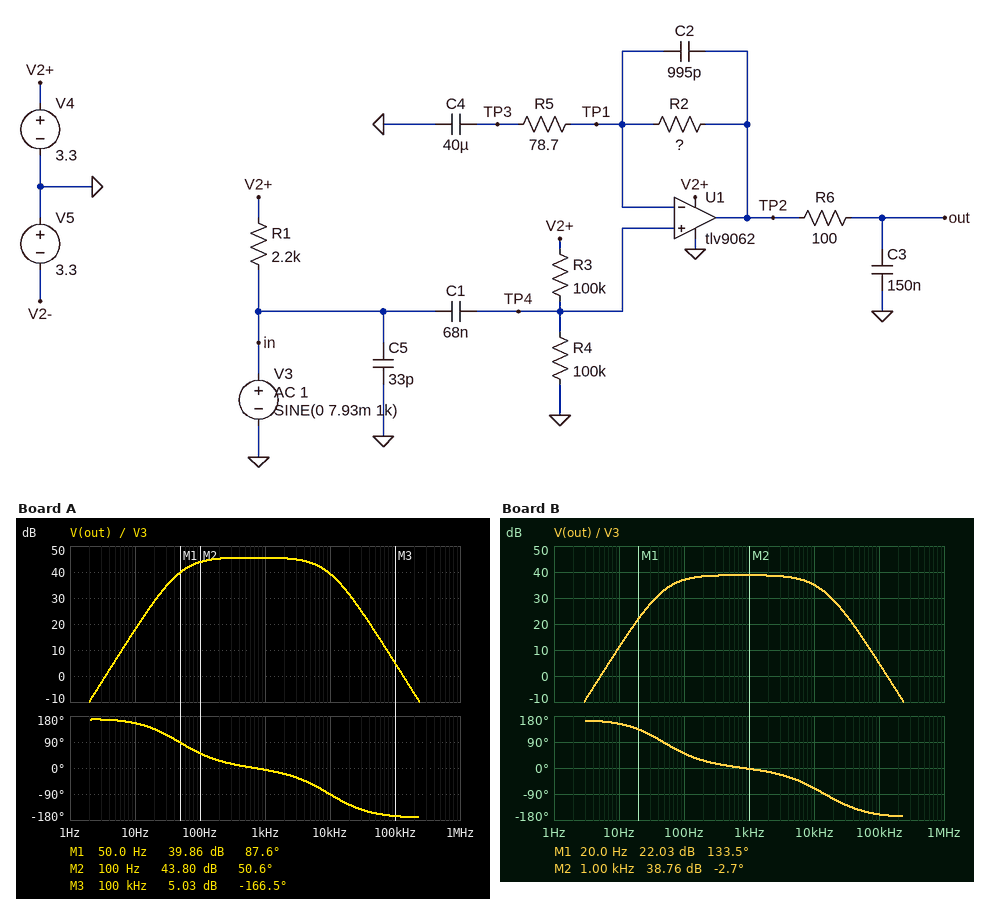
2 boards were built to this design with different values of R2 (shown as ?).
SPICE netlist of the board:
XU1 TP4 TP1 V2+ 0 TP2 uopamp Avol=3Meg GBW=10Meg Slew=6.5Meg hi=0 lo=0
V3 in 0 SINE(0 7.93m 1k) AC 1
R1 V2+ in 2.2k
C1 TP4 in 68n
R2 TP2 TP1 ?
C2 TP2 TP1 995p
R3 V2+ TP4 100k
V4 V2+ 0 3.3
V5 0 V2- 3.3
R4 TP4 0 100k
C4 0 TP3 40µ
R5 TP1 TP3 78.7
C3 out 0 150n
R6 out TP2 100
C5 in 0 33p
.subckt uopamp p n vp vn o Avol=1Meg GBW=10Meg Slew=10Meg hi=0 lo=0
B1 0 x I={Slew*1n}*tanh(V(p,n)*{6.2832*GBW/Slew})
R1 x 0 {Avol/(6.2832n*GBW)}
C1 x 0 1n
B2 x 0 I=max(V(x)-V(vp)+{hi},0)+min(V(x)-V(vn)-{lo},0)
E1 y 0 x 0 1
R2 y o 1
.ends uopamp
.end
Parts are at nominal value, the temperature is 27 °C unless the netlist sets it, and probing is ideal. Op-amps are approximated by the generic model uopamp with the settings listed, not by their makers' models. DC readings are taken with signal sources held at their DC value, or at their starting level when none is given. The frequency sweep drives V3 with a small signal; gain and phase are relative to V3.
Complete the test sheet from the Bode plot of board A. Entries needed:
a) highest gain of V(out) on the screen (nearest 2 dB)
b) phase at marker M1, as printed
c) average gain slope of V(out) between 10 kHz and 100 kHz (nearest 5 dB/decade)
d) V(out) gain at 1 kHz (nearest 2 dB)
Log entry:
46 dB
87.6 deg
-35 dB/decade
46 dB
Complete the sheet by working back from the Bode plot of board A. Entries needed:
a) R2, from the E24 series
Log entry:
15 kΩ
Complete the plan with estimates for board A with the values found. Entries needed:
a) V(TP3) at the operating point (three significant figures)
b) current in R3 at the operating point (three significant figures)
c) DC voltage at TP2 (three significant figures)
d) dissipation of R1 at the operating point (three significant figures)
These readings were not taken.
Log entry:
1.65 V
16.5 µA
1.65 V
4.95 mW
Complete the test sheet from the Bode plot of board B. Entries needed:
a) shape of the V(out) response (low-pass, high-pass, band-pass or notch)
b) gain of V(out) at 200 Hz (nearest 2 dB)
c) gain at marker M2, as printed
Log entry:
band-pass
38 dB
38.76 dB
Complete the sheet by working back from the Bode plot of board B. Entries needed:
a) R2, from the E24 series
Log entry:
6.8 kΩ
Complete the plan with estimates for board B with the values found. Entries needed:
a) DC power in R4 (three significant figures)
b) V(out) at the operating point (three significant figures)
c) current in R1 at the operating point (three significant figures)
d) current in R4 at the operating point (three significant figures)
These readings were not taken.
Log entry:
27.2 µW
1.65 V
1.50 mA
16.5 µA
